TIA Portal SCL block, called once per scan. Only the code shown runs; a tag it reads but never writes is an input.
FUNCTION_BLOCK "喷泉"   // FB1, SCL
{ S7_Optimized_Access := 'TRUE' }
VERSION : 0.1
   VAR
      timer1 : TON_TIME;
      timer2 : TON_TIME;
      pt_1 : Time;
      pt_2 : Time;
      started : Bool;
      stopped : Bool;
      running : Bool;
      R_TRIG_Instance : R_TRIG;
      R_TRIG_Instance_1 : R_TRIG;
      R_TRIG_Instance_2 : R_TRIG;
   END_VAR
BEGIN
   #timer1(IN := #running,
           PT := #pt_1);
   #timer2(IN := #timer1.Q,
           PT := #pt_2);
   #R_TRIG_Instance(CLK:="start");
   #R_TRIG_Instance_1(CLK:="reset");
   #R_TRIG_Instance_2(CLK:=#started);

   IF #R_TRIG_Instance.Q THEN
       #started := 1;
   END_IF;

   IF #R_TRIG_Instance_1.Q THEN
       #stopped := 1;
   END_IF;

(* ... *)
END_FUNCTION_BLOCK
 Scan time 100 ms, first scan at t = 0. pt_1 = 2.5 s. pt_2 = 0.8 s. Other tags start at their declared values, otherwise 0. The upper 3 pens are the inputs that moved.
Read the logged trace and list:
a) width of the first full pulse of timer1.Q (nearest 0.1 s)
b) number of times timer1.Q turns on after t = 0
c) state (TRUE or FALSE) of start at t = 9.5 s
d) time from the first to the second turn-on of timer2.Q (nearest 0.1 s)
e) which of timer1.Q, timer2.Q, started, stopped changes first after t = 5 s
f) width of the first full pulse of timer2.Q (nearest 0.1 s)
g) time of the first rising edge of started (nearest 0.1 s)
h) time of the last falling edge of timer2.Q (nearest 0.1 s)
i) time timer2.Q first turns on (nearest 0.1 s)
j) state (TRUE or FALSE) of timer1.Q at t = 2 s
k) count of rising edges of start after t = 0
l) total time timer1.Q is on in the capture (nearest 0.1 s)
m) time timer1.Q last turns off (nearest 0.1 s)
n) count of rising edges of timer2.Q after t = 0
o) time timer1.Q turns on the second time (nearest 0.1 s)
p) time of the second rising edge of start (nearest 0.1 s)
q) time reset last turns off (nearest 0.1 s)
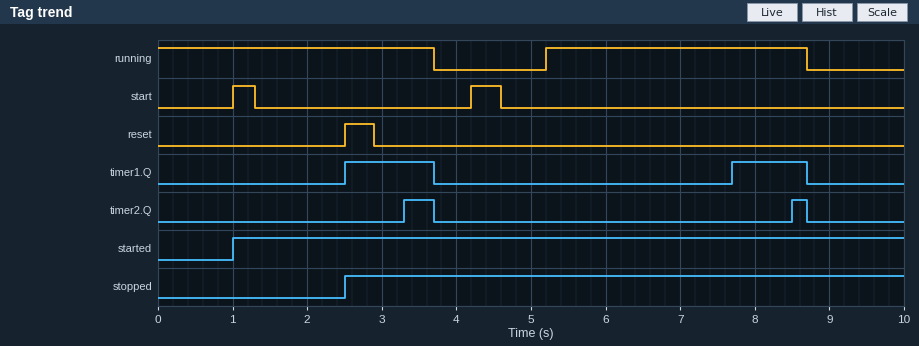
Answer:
1.2 s
2
FALSE
5.2 s
timer1.Q
0.4 s
1.0 s
8.7 s
3.3 s
FALSE
2
2.2 s
8.7 s
2
7.7 s
4.2 s
2.9 s
